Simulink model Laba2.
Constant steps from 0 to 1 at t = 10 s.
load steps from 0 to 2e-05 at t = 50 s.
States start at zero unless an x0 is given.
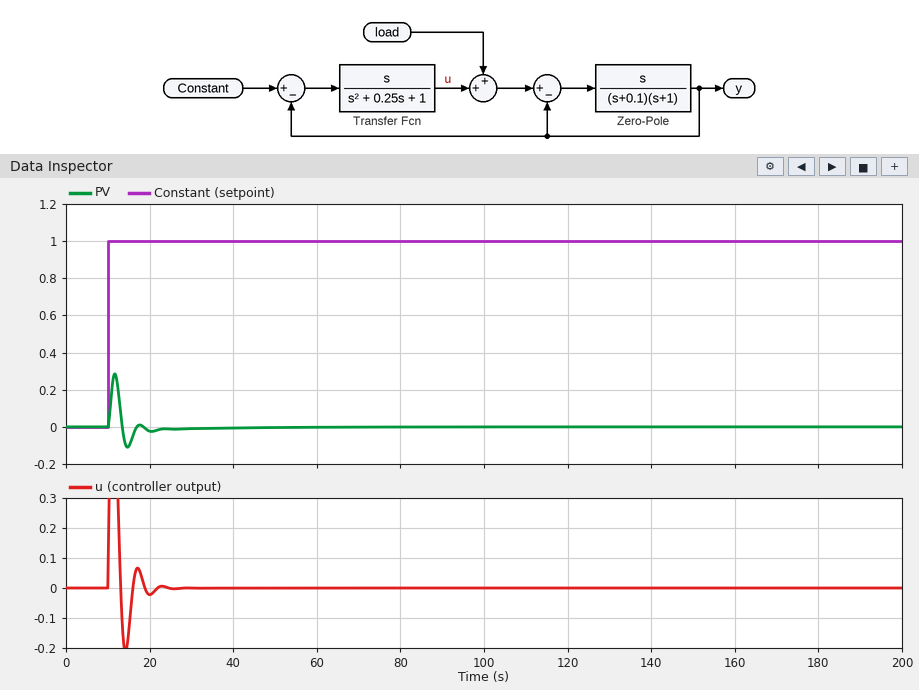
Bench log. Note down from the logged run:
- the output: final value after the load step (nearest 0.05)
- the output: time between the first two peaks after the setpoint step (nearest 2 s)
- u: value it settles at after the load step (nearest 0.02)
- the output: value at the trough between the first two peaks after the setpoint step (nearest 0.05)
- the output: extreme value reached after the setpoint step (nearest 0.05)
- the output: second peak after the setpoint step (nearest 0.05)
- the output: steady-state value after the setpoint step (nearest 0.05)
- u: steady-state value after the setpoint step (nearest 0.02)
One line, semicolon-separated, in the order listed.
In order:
0.00; 6 s; 0.00; -0.10; 0.30; 0.00; 0.00; 0.00
